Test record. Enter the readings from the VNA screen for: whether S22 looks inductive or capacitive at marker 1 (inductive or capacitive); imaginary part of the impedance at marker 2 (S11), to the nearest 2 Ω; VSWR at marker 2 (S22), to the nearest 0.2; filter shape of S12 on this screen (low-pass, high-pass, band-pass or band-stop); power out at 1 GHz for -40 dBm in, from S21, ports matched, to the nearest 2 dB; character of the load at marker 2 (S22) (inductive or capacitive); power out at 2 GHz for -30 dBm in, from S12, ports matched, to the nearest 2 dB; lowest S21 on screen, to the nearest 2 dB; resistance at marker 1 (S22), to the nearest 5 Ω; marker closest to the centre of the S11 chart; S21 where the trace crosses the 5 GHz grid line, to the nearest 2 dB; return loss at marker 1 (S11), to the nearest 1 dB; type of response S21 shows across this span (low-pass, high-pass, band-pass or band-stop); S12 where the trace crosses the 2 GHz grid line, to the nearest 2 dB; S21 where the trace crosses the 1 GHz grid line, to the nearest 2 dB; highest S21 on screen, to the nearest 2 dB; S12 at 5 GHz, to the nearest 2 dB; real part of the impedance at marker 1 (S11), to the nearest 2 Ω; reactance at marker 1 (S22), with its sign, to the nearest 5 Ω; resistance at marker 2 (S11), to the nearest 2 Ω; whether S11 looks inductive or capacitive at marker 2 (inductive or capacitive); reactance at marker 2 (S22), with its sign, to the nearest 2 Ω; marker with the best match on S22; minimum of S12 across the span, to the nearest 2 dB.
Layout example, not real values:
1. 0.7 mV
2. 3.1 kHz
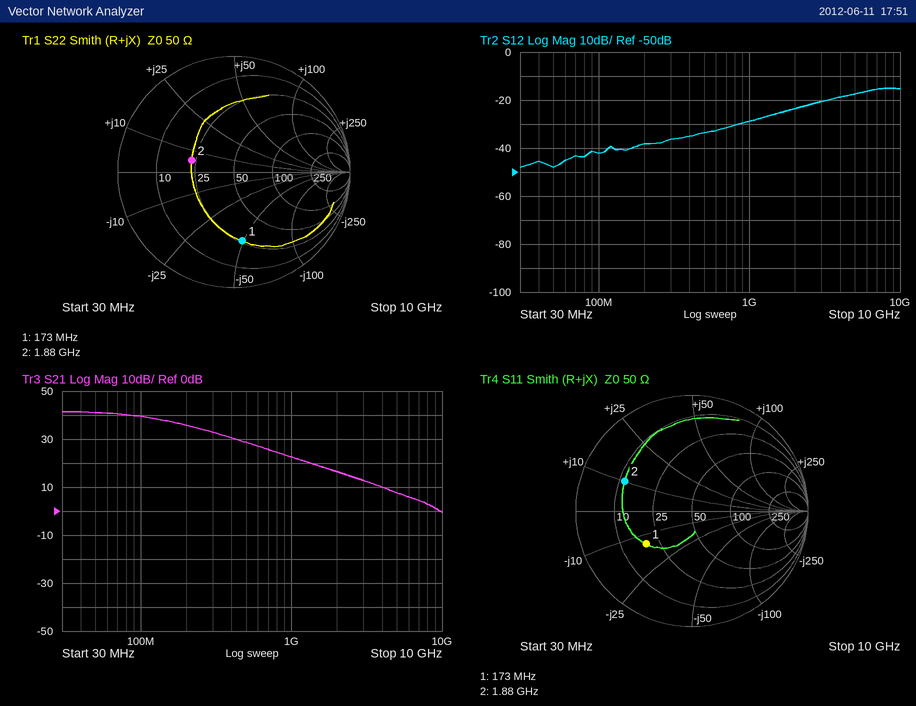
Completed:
1. capacitive
2. +10 Ω
3. 2.2
4. high-pass
5. -18 dBm
6. inductive
7. -54 dBm
8. 0 dB
9. 25 Ω
10. marker 1
11. 8 dB
12. 6 dB
13. low-pass
14. -24 dB
15. 22 dB
16. 42 dB
17. -18 dB
18. 18 Ω
19. -50 Ω
20. 12 Ω
21. inductive
22. +6 Ω
23. marker 2
24. -48 dB
